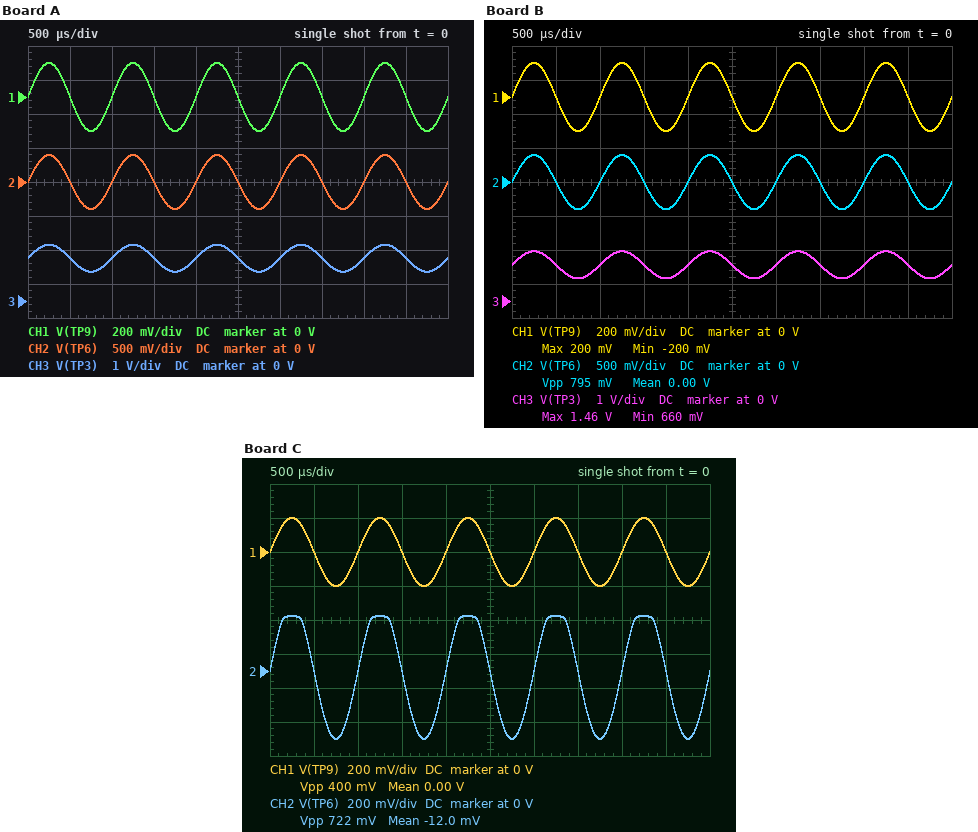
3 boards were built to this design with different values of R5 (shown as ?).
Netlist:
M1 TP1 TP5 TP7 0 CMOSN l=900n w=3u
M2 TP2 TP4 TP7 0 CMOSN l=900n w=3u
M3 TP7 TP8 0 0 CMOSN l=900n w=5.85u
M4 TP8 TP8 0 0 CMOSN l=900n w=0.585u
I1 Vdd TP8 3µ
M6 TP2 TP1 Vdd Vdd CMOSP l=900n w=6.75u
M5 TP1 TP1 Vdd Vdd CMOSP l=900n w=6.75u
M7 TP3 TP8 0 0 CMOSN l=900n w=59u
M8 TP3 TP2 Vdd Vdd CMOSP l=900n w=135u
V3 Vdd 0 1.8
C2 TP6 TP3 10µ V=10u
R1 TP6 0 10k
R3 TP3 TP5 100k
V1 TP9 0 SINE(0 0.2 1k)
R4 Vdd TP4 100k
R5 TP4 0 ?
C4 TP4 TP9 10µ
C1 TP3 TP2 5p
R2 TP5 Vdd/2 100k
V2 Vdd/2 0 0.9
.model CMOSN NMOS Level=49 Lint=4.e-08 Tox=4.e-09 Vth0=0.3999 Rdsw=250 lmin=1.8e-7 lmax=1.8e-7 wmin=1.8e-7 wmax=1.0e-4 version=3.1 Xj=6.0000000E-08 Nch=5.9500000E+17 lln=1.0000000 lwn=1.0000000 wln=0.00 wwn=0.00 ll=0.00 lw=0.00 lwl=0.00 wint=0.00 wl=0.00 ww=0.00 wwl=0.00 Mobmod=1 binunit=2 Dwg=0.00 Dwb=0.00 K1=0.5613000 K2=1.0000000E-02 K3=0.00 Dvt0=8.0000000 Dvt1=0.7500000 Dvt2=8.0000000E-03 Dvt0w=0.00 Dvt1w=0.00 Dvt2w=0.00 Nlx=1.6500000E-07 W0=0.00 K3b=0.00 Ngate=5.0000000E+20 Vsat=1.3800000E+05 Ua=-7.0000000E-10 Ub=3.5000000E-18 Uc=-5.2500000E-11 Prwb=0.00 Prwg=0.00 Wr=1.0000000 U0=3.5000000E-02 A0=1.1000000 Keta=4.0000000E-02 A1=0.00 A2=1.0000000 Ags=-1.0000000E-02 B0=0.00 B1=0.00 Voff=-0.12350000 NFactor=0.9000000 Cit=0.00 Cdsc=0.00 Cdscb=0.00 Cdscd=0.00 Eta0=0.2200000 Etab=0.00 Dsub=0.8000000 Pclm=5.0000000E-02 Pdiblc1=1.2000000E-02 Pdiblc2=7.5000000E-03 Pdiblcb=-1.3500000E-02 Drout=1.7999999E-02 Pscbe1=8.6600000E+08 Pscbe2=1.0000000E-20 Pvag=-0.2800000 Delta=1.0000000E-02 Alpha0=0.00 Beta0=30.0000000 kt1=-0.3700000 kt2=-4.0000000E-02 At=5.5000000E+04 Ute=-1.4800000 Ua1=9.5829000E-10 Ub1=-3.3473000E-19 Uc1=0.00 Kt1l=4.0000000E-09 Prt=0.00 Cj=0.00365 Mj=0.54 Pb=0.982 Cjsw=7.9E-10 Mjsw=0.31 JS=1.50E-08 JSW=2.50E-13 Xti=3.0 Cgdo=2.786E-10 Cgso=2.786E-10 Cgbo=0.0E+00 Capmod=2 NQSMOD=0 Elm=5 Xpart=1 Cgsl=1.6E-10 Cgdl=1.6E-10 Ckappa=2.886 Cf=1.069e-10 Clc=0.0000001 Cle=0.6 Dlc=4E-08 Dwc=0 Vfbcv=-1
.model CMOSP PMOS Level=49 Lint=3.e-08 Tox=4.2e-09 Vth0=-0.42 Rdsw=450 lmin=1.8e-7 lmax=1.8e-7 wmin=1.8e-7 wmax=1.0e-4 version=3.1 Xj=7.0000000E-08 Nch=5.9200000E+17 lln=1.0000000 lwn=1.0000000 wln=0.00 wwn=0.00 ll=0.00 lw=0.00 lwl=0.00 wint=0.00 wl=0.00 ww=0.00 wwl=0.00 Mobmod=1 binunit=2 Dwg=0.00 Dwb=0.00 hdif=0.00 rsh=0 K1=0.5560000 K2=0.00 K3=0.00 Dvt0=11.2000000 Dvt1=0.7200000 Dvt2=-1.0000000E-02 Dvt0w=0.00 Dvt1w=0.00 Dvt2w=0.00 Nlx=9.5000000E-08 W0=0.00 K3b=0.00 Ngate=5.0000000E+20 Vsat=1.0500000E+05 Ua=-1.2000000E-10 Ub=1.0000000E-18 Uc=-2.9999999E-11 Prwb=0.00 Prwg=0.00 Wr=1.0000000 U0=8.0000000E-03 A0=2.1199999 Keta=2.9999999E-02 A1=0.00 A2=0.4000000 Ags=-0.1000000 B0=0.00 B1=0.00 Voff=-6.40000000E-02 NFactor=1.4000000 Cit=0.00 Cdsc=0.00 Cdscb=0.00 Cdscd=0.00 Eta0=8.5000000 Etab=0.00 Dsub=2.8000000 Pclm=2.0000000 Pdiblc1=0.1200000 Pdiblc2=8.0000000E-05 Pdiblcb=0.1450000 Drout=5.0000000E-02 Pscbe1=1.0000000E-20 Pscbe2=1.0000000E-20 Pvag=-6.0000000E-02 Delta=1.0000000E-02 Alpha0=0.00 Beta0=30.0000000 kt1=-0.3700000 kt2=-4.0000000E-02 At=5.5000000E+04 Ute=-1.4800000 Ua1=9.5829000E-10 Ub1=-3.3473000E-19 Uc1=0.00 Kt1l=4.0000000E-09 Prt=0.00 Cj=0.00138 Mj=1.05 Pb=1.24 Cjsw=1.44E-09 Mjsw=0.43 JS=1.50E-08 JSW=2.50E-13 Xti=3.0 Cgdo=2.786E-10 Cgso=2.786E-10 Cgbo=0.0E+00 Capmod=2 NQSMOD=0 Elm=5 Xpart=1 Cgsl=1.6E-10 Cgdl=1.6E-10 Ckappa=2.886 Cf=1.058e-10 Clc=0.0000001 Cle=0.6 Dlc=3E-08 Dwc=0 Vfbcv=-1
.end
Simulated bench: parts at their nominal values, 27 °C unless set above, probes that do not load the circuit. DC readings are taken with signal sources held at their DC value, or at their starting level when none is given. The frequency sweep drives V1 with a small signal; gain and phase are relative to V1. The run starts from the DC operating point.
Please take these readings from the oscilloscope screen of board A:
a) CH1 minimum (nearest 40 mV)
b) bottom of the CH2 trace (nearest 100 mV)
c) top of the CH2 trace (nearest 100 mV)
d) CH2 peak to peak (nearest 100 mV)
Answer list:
-200 mV
-400 mV
400 mV
800 mV
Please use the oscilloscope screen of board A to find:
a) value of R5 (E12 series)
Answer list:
150 kΩ
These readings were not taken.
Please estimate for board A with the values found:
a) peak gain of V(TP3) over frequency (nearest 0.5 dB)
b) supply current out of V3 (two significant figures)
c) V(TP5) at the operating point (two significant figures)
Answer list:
6.0 dB
360 µA
1.1 V
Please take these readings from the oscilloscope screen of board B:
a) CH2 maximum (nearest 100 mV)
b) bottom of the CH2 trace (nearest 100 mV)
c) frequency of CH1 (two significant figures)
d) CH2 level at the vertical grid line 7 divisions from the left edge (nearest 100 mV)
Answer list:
400 mV
-400 mV
1.0 kHz
0 V
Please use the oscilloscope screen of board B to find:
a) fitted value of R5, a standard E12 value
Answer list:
120 kΩ
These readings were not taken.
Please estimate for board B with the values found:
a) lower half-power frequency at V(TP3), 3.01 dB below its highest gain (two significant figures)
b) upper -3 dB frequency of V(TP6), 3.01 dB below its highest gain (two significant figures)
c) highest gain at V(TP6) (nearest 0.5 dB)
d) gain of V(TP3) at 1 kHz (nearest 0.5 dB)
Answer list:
290 mHz
2.1 MHz
6.0 dB
6.0 dB
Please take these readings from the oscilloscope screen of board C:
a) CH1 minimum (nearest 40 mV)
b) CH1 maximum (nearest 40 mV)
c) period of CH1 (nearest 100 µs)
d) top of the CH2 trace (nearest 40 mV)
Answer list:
-200 mV
200 mV
1.0 ms
320 mV
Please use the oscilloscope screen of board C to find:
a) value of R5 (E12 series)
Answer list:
180 kΩ
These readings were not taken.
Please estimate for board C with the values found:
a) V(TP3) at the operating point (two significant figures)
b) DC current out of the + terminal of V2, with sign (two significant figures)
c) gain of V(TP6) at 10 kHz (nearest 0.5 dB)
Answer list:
1.4 V
-2.6 µA
6.0 dB
